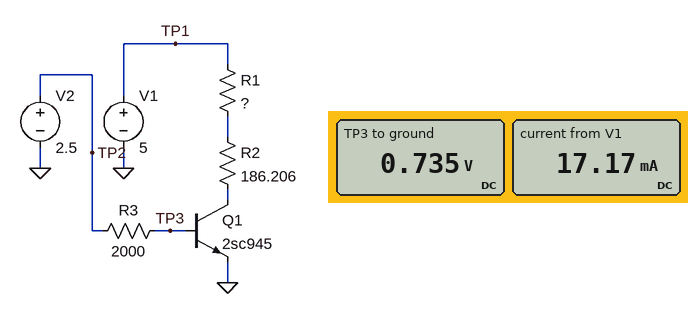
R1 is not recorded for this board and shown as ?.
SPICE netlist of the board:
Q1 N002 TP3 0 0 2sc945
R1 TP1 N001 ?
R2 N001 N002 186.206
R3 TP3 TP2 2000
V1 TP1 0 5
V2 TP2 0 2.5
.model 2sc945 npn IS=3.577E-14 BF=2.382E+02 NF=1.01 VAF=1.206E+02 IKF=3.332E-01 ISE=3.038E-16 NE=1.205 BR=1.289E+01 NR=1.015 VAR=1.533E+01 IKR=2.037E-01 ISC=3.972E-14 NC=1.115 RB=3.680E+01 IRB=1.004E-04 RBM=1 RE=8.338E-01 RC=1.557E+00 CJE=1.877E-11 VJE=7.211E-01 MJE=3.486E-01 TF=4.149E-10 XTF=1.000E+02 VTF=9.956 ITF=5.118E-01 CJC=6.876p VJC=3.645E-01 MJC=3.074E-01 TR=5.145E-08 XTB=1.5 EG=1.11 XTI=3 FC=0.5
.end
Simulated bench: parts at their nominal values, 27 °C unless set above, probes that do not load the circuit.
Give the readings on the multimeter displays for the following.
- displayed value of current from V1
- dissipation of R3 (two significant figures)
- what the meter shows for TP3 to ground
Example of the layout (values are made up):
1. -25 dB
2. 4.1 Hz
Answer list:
1. 17.17 mA
2. 1.6 mW
3. 0.735 V
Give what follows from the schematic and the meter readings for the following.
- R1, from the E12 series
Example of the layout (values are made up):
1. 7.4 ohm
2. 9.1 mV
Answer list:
1. 100 Ω
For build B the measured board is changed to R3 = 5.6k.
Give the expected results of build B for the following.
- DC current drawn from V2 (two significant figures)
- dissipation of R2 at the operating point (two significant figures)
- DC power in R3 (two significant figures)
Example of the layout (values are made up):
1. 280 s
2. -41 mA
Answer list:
1. 320 µA
2. 54 mW
3. 560 µW
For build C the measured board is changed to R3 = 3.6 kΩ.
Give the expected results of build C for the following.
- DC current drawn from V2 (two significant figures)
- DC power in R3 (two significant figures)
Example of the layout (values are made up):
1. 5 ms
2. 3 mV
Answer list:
1. 490 µA
2. 870 µW
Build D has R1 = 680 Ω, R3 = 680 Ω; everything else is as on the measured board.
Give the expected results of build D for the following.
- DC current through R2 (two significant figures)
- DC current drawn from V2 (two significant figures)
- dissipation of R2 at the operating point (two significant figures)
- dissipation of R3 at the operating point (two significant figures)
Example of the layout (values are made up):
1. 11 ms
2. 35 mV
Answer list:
1. 5.7 mA
2. 2.6 mA
3. 6.1 mW
4. 4.6 mW
